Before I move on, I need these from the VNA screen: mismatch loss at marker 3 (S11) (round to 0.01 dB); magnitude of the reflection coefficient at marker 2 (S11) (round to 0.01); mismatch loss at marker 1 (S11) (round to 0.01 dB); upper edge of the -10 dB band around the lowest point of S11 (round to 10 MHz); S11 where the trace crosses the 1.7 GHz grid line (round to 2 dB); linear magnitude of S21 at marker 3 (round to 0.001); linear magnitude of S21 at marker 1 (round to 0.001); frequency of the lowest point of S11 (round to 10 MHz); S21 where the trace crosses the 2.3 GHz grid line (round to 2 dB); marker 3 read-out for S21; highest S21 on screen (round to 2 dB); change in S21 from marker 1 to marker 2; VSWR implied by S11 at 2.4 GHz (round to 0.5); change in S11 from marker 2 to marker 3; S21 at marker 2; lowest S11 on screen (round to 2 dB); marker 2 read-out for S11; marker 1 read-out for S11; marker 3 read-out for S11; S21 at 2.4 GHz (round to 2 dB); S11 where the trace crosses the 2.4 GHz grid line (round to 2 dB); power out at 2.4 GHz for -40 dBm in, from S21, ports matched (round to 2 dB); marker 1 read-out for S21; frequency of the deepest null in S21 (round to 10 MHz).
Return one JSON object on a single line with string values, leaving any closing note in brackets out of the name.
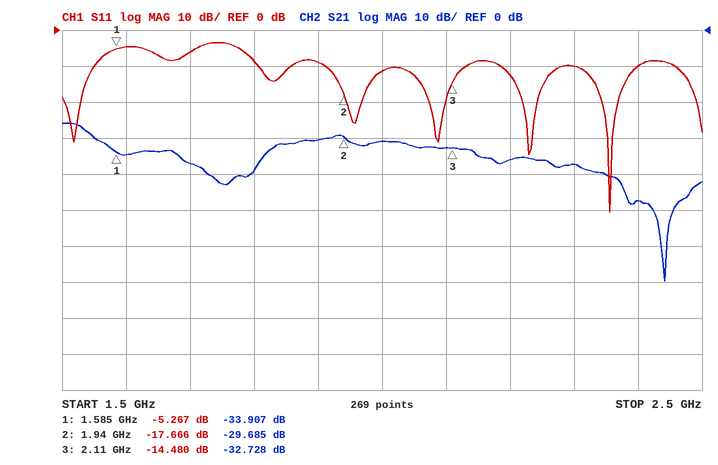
{"mismatch loss at marker 3 (S11)": "0.16 dB", "magnitude of the reflection coefficient at marker 2 (S11)": "0.13", "mismatch loss at marker 1 (S11)": "1.53 dB", "upper edge of the -10 dB band around the lowest point of S11": "2.40 GHz", "S11 where the trace crosses the 1.7 GHz grid line": "-6 dB", "linear magnitude of S21 at marker 3": "0.023", "linear magnitude of S21 at marker 1": "0.020", "frequency of the lowest point of S11": "2.36 GHz", "S21 where the trace crosses the 2.3 GHz grid line": "-38 dB", "marker 3 read-out for S21": "-32.728 dB", "highest S21 on screen": "-26 dB", "change in S21 from marker 1 to marker 2": "4.222 dB", "VSWR implied by S11 at 2.4 GHz": "2.0", "change in S11 from marker 2 to marker 3": "3.186 dB", "S21 at marker 2": "-29.685 dB", "lowest S11 on screen": "-50 dB", "marker 2 read-out for S11": "-17.666 dB", "marker 1 read-out for S11": "-5.267 dB", "marker 3 read-out for S11": "-14.480 dB", "S21 at 2.4 GHz": "-48 dB", "S11 where the trace crosses the 2.4 GHz grid line": "-10 dB", "power out at 2.4 GHz for -40 dBm in, from S21, ports matched": "-88 dBm", "marker 1 read-out for S21": "-33.907 dB", "frequency of the deepest null in S21": "2.44 GHz"}
